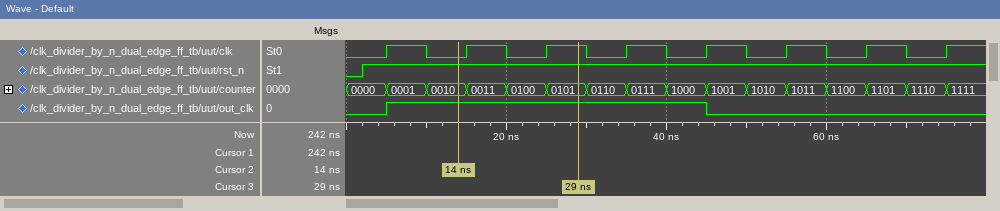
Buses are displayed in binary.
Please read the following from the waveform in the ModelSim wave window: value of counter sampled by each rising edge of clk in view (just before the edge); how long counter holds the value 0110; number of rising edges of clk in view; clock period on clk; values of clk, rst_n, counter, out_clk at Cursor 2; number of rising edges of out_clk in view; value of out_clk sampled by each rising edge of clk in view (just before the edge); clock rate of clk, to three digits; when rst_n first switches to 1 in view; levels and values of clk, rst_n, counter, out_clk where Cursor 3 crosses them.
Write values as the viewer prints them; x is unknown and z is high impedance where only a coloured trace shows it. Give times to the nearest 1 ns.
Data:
0000, 0010, 0100, 0110, 1000, 1010, 1100, 1110
5 ns
8
10 ns
clk=0, rst_n=1, counter=0010, out_clk=1
1
0 1 1 1 1 0 0 0
100 MHz
2 ns
clk=1, rst_n=1, counter=0101, out_clk=1
